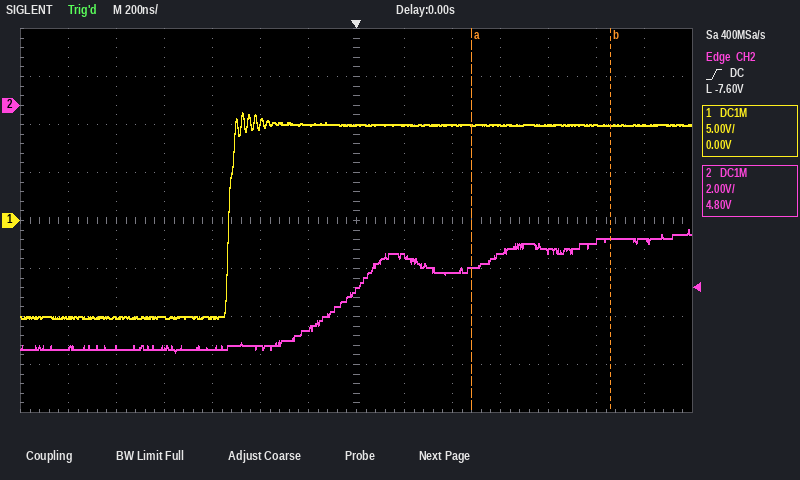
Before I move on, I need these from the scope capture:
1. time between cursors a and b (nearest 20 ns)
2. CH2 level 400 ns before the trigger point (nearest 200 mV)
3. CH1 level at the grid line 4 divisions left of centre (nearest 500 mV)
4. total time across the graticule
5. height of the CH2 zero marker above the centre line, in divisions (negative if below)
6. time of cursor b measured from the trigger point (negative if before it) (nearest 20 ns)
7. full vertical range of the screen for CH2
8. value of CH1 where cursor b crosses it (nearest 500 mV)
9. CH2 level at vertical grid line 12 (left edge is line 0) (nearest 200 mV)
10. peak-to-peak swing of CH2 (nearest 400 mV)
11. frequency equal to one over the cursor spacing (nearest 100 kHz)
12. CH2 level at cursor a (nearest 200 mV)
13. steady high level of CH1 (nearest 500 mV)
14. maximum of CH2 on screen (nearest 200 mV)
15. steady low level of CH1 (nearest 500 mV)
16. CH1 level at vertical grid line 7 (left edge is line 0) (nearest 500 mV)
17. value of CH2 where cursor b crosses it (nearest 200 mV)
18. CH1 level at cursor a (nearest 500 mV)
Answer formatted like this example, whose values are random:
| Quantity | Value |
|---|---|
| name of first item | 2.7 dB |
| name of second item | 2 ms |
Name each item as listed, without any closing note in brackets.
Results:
| Quantity | Value |
|---|---|
| time between cursors a and b | 580 ns |
| CH2 level 400 ns before the trigger point | -10.0 V |
| CH1 level at the grid line 4 divisions left of centre | -10.0 V |
| total time across the graticule | 2.8 µs |
| height of the CH2 zero marker above the centre line, in divisions | +2.4 div |
| time of cursor b measured from the trigger point (negative if before it) | +1.06 µs |
| full vertical range of the screen for CH2 | 16 V |
| value of CH1 where cursor b crosses it | 10.0 V |
| CH2 level at vertical grid line 12 (left edge is line 0) | -5.6 V |
| peak-to-peak swing of CH2 | 5.2 V |
| frequency equal to one over the cursor spacing | 1.7 MHz |
| CH2 level at cursor a | -6.8 V |
| steady high level of CH1 | 10.0 V |
| maximum of CH2 on screen | -5.2 V |
| steady low level of CH1 | -10.0 V |
| CH1 level at vertical grid line 7 (left edge is line 0) | 10.0 V |
| value of CH2 where cursor b crosses it | -5.6 V |
| CH1 level at cursor a | 10.0 V |
